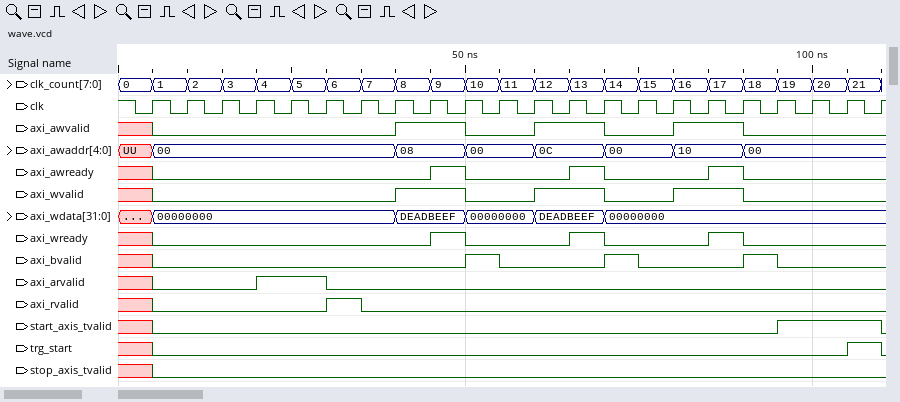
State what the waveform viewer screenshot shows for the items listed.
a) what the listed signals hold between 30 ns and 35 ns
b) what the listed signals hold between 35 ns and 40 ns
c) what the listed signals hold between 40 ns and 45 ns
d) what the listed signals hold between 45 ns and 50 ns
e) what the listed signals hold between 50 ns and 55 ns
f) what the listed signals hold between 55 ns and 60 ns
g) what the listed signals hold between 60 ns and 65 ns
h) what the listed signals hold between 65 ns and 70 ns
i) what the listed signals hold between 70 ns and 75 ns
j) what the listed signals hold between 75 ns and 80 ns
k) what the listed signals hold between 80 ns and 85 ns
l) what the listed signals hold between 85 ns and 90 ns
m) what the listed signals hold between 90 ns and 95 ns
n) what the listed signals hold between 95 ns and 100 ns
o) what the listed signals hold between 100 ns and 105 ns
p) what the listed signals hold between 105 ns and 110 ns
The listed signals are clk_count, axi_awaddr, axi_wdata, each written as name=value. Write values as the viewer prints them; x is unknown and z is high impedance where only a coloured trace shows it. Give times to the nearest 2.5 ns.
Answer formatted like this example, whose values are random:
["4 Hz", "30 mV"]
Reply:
["clk_count=6, axi_awaddr=00, axi_wdata=00000000", "clk_count=7, axi_awaddr=00, axi_wdata=00000000", "clk_count=8, axi_awaddr=08, axi_wdata=DEADBEEF", "clk_count=9, axi_awaddr=08, axi_wdata=DEADBEEF", "clk_count=10, axi_awaddr=00, axi_wdata=00000000", "clk_count=11, axi_awaddr=00, axi_wdata=00000000", "clk_count=12, axi_awaddr=0C, axi_wdata=DEADBEEF", "clk_count=13, axi_awaddr=0C, axi_wdata=DEADBEEF", "clk_count=14, axi_awaddr=00, axi_wdata=00000000", "clk_count=15, axi_awaddr=00, axi_wdata=00000000", "clk_count=16, axi_awaddr=10, axi_wdata=00000000", "clk_count=17, axi_awaddr=10, axi_wdata=00000000", "clk_count=18, axi_awaddr=00, axi_wdata=00000000", "clk_count=19, axi_awaddr=00, axi_wdata=00000000", "clk_count=20, axi_awaddr=00, axi_wdata=00000000", "clk_count=21, axi_awaddr=00, axi_wdata=00000000"]
